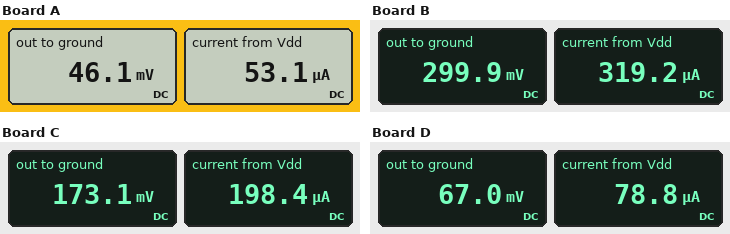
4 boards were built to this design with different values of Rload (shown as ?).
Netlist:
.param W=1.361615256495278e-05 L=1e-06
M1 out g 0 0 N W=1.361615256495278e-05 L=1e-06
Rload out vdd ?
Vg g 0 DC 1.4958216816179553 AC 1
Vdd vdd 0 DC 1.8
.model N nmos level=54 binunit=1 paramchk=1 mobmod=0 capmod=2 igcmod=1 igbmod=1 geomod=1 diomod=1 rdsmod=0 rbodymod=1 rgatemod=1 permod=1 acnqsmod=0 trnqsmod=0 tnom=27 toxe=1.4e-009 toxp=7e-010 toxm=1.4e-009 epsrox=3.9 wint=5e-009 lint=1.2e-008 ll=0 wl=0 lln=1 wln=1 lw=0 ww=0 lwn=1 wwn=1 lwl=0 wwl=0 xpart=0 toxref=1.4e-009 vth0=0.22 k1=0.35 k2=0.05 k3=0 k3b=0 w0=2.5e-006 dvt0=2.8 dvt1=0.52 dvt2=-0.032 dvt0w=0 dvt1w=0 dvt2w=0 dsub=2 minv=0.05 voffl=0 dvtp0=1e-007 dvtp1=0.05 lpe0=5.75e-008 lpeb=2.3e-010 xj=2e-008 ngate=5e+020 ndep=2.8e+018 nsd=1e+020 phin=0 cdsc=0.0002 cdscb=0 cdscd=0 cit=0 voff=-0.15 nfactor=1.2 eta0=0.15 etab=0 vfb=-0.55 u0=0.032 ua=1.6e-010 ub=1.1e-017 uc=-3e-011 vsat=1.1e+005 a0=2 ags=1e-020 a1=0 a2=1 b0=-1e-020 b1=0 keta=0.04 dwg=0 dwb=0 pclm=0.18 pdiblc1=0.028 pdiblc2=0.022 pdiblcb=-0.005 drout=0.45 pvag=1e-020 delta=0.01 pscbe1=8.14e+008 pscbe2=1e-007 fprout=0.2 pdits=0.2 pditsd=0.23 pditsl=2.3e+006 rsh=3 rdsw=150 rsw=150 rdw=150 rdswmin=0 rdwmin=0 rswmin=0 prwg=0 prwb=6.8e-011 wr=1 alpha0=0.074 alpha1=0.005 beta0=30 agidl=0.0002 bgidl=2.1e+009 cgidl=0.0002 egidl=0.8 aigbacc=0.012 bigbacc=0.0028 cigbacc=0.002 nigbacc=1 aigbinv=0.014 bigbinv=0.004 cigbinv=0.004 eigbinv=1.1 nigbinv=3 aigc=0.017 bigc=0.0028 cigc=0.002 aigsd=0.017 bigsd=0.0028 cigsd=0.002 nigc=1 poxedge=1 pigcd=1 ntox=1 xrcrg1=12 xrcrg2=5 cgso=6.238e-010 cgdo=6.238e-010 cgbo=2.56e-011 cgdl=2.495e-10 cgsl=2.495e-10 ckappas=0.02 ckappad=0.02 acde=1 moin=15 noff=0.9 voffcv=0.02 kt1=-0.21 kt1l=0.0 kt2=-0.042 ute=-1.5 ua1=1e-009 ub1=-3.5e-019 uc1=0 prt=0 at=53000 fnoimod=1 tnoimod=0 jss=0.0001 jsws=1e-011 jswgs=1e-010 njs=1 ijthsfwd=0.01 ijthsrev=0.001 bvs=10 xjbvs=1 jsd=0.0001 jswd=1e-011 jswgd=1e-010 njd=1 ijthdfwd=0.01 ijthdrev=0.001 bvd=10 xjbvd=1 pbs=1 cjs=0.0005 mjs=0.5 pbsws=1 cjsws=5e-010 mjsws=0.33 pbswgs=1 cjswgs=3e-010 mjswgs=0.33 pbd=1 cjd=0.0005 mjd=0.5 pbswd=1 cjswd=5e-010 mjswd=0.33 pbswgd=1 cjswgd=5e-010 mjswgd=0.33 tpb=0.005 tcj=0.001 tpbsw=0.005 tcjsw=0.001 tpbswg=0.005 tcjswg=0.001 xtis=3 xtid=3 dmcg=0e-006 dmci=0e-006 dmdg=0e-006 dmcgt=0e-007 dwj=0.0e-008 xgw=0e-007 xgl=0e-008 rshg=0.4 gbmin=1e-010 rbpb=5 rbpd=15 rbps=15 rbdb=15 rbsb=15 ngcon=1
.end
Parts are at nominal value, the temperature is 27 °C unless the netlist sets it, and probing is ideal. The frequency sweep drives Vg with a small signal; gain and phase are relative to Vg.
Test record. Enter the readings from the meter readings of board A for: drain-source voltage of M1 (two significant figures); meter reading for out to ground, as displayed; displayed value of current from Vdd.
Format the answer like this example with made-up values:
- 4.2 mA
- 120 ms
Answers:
- 46 mV
- 46.1 mV
- 53.1 µA
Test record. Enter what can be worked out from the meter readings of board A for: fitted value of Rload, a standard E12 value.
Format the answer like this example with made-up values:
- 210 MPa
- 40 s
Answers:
- 33 kΩ
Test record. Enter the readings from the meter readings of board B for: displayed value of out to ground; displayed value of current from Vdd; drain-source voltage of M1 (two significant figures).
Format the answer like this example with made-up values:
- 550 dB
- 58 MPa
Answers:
- 299.9 mV
- 319.2 µA
- 300 mV
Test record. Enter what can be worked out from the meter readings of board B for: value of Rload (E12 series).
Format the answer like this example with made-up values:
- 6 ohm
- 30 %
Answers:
- 4.7 kΩ
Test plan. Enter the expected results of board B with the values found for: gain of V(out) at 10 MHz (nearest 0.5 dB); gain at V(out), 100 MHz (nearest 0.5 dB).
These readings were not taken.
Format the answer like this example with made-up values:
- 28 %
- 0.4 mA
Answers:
- -29.5 dB
- -16.0 dB
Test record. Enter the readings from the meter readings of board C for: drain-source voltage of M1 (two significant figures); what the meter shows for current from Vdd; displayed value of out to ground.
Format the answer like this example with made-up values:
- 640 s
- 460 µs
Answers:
- 170 mV
- 198.4 µA
- 173.1 mV
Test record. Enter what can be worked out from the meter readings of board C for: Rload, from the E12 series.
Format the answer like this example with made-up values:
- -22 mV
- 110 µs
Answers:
- 8.2 kΩ
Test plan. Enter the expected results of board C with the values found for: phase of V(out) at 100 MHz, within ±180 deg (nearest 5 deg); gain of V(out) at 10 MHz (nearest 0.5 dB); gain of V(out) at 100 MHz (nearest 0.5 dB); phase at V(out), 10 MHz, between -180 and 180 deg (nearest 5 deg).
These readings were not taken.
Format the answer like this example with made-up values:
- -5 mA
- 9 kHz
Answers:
- 65 deg
- -28.0 dB
- -16.5 dB
- 20 deg
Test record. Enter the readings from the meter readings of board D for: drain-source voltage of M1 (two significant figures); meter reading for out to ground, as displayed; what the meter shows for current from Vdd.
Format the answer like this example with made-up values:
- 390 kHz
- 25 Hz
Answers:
- 67 mV
- 67.0 mV
- 78.8 µA
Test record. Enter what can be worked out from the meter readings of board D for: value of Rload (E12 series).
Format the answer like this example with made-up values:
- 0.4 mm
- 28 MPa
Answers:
- 22 kΩ
